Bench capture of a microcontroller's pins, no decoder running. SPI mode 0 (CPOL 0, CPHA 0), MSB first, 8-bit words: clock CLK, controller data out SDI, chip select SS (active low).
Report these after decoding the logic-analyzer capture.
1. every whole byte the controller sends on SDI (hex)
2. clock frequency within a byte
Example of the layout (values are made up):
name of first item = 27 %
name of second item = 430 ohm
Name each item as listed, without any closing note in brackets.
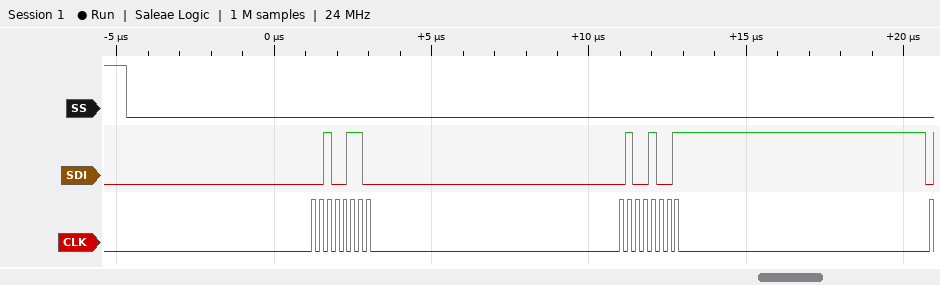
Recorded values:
every whole byte the controller sends on SDI = 26 49
clock frequency within a byte = 4 MHz
